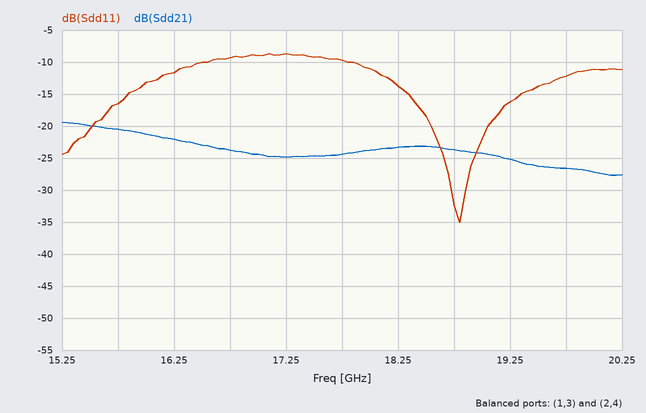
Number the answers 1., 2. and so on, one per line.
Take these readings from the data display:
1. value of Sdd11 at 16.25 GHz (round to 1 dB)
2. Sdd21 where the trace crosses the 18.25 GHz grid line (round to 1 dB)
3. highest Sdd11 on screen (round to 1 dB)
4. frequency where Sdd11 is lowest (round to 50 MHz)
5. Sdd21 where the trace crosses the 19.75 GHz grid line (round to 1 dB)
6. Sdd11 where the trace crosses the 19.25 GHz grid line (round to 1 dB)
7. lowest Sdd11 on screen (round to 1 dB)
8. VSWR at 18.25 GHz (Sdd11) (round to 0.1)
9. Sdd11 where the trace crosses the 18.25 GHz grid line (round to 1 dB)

1. -12 dB
2. -23 dB
3. -9 dB
4. 18.80 GHz
5. -27 dB
6. -16 dB
7. -35 dB
8. 1.5
9. -14 dB
